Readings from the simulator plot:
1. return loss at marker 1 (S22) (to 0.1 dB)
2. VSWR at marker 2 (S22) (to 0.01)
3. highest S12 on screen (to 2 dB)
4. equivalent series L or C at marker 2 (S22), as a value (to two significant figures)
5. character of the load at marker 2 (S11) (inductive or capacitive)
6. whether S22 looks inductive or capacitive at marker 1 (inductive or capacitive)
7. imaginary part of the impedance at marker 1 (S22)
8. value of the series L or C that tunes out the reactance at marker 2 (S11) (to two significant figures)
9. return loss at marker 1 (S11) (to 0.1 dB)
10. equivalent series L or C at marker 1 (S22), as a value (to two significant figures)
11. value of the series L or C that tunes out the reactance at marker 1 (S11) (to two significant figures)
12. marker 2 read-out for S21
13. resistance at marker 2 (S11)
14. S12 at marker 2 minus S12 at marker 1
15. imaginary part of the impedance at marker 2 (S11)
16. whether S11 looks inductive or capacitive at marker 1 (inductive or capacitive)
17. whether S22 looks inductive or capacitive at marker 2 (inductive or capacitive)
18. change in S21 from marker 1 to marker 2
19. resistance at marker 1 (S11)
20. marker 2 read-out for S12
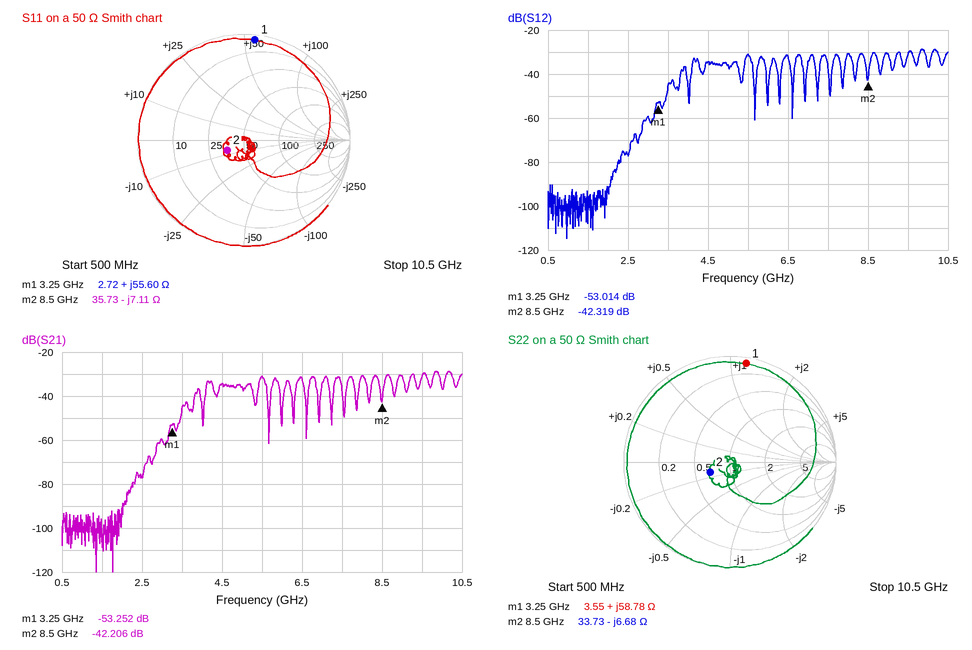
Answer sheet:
0.5 dB
1.53
-28 dB
2.8 pF
capacitive
inductive
+58.78 Ω
130 pH
0.4 dB
2.9 nH
880 fF
-42.206 dB
35.73 Ω
10.695 dB
-7.11 Ω
inductive
capacitive
11.046 dB
2.72 Ω
-42.319 dB
